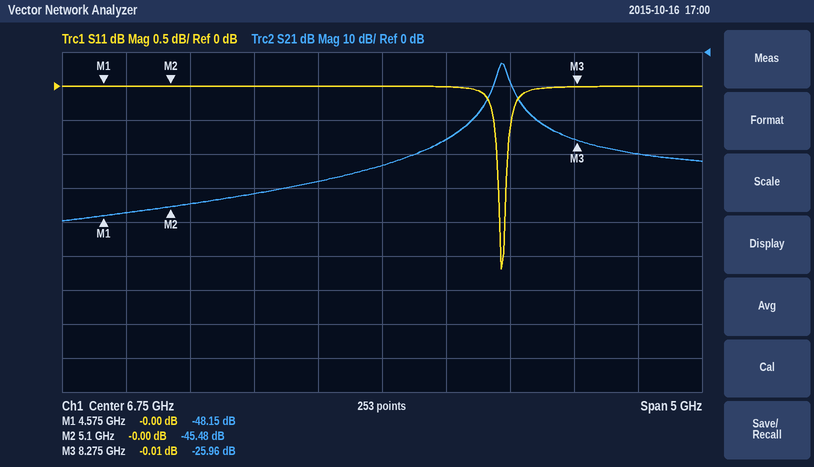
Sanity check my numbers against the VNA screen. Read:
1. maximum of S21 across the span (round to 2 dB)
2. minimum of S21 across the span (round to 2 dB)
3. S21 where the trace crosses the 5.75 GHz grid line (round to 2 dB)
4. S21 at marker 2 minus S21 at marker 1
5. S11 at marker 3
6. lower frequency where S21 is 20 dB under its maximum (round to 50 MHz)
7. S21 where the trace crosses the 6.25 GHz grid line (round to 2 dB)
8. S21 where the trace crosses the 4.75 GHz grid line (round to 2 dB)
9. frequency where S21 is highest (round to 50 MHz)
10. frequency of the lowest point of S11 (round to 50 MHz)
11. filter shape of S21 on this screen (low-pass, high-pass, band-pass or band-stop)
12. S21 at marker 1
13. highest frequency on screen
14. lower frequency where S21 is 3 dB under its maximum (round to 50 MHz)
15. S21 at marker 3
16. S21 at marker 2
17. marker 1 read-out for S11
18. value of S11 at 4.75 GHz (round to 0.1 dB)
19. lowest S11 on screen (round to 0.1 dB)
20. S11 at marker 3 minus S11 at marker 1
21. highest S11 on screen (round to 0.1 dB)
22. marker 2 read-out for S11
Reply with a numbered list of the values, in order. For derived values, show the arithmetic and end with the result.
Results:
1. -4 dB
2. -50 dB
3. -42 dB
4. -45.48 − (-48.15) = 2.67 dB
5. -0.01 dB
6. 7.35 GHz
7. -38 dB
8. -48 dB
9. 7.70 GHz
10. 7.70 GHz
11. band-pass
12. -48.15 dB
13. 9.25 GHz
14. 7.65 GHz
15. -25.96 dB
16. -45.48 dB
17. -0.00 dB
18. 0.0 dB
19. -2.7 dB
20. -0.01 − (-0) = -0.01 dB
21. 0.0 dB
22. -0.00 dB
